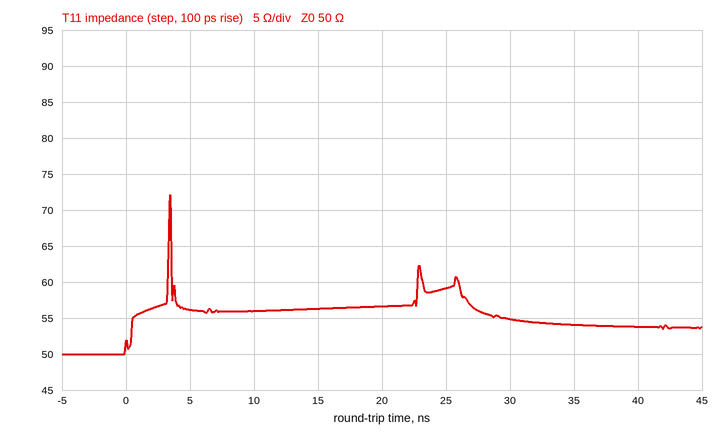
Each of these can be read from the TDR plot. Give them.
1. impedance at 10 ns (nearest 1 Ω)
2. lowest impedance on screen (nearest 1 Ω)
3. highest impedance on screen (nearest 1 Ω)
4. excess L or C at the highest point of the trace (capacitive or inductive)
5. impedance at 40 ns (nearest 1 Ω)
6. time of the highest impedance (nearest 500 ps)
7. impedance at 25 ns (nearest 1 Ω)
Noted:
56 Ω
50 Ω
72 Ω
inductive
54 Ω
3.5 ns
59 Ω
